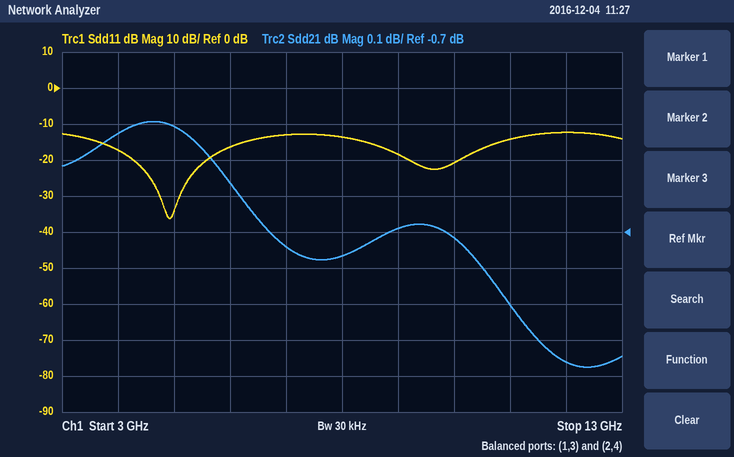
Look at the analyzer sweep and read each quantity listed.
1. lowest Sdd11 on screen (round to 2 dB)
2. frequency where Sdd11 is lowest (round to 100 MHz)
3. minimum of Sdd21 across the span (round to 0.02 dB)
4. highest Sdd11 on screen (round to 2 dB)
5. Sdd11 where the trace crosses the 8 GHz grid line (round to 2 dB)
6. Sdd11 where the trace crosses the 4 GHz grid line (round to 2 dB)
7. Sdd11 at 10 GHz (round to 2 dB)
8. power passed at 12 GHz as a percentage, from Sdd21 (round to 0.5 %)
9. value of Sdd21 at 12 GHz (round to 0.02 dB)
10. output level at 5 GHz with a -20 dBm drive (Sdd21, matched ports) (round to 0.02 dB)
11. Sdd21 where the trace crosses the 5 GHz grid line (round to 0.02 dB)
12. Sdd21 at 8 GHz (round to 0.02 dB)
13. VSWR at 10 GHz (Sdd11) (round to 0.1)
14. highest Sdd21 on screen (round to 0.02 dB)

-36 dB
4.9 GHz
-1.08 dB
-12 dB
-14 dB
-18 dB
-20 dB
78.5 %
-1.06 dB
-20.40 dBm
-0.40 dB
-0.76 dB
1.2
-0.40 dB
